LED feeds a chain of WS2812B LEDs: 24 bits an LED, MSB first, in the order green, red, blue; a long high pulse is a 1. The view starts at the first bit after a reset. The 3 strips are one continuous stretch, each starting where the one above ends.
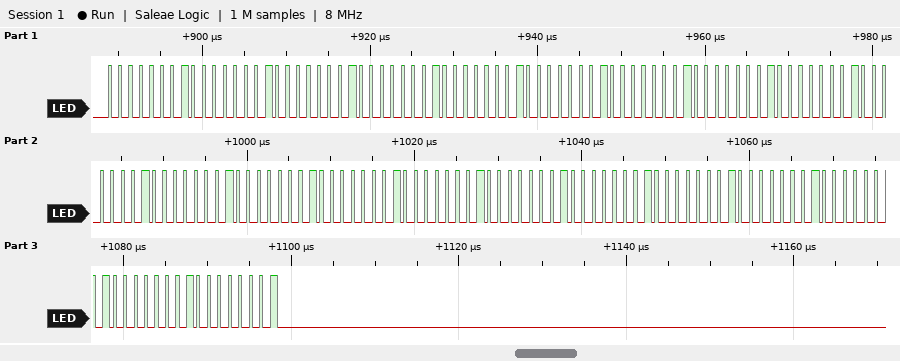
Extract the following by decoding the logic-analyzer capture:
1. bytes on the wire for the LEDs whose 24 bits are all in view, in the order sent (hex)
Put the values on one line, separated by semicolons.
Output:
01 01 01 01 01 01 01 01 01 01 01 01 01 01 01 01 01 01 01 01 01
